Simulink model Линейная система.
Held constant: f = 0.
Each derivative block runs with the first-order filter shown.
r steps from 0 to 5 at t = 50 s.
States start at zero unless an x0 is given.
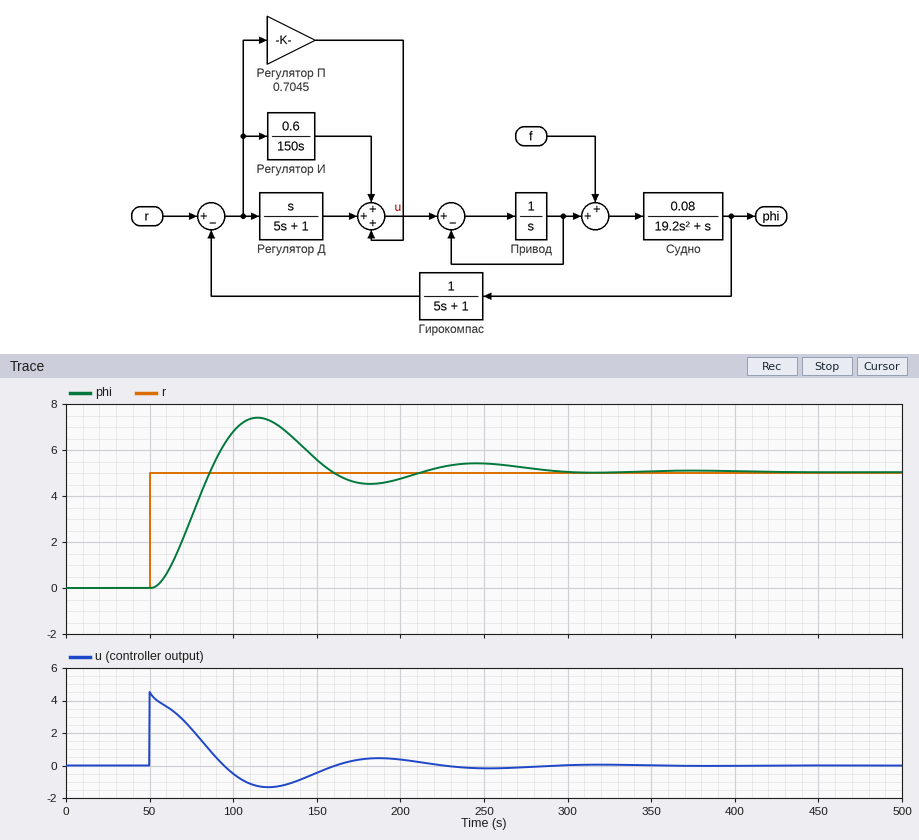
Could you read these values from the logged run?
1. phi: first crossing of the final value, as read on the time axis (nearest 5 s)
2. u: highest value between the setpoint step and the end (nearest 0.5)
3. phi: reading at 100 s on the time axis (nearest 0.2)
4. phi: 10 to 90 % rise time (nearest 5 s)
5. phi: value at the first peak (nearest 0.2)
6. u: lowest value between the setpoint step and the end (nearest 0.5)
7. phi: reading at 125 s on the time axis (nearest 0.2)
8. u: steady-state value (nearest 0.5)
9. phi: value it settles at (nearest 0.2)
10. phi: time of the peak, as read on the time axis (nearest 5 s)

85 s
4.5
6.8
25 s
7.4
-1.5
7.2
0.0
5.0
115 s
